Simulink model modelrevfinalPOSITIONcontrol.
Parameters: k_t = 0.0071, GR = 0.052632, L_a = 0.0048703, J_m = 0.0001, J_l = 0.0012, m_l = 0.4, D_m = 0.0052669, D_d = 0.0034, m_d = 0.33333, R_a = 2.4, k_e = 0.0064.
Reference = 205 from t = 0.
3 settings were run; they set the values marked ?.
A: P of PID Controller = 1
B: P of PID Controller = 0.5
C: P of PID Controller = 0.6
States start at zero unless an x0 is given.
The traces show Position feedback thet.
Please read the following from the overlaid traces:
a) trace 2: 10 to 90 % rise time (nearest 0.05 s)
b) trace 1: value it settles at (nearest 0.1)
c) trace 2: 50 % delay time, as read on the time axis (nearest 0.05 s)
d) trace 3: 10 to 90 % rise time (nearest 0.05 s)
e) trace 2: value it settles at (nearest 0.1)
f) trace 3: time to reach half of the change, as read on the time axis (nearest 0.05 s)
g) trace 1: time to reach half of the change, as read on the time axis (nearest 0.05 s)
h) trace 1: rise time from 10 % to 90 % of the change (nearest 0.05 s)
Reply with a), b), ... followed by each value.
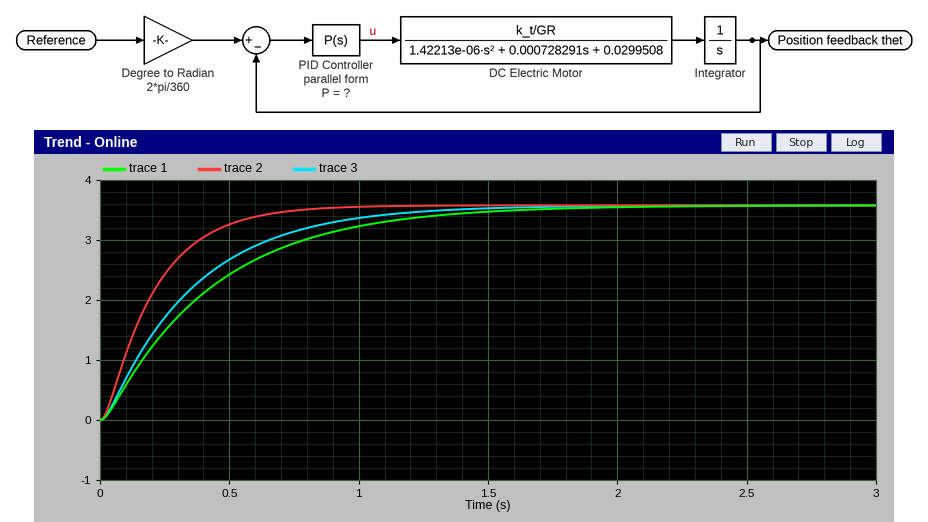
a) 0.45 s
b) 3.6
c) 0.15 s
d) 0.75 s
e) 3.6
f) 0.25 s
g) 0.30 s
h) 0.90 s
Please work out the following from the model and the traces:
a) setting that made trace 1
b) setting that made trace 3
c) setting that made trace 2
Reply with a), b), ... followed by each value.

a) B
b) C
c) A
